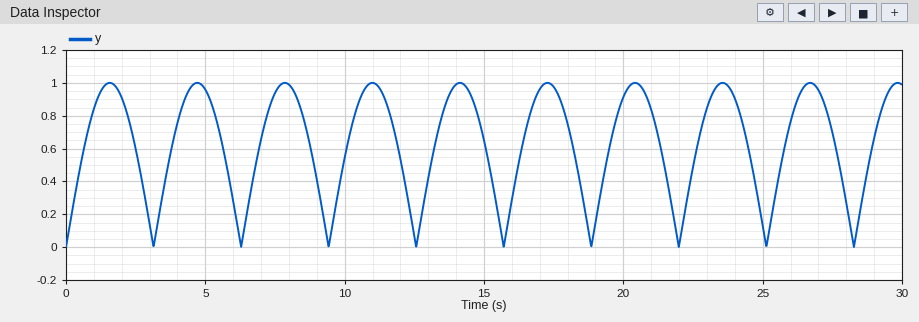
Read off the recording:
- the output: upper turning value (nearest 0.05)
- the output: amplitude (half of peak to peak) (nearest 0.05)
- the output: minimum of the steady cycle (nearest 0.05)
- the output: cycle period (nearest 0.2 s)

1.00
0.50
0.00
3.2 s
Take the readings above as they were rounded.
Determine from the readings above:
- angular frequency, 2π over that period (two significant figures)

2.0 rad/s
